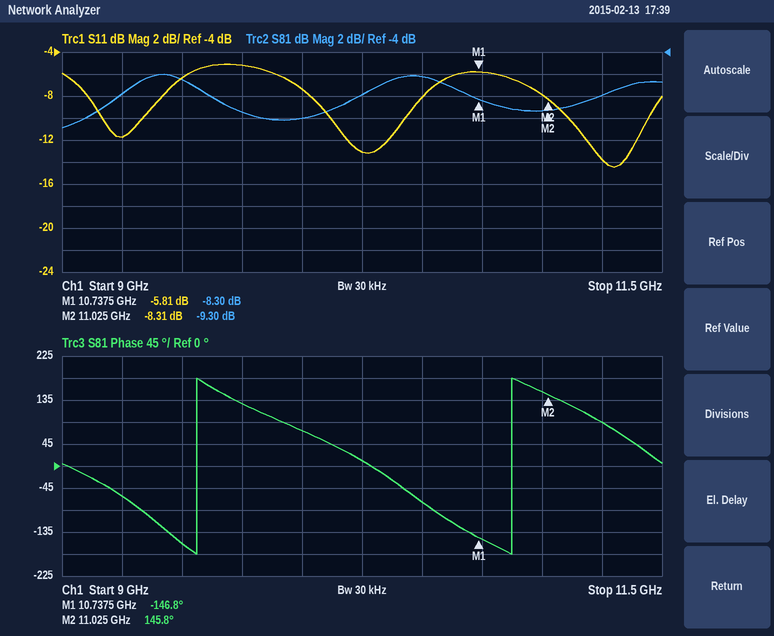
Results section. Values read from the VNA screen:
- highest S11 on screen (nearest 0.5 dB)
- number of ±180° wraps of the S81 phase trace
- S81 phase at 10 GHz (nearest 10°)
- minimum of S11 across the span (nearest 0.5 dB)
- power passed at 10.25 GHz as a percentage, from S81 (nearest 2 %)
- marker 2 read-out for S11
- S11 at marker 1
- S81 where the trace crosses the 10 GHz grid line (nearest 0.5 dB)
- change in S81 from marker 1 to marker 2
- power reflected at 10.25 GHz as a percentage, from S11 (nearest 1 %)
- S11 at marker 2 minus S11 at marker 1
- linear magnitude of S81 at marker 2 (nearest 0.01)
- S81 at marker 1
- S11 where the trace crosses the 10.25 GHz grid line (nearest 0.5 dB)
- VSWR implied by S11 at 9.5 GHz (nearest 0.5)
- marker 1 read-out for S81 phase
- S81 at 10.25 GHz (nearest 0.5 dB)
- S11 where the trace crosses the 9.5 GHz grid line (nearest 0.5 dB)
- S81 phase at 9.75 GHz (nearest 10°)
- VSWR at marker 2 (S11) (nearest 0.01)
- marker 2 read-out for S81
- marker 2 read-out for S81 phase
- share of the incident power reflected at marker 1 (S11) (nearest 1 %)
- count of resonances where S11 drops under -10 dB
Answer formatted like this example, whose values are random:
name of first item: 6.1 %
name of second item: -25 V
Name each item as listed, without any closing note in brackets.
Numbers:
highest S11 on screen: -5.0 dB
number of ±180° wraps of the S81 phase trace: 2
S81 phase at 10 GHz: 70°
minimum of S11 across the span: -14.5 dB
power passed at 10.25 GHz as a percentage, from S81: 16 %
marker 2 read-out for S11: -8.31 dB
S11 at marker 1: -5.81 dB
S81 where the trace crosses the 10 GHz grid line: -10.0 dB
change in S81 from marker 1 to marker 2: -1.00 dB
power reflected at 10.25 GHz as a percentage, from S11: 5 %
S11 at marker 2 minus S11 at marker 1: -2.50 dB
linear magnitude of S81 at marker 2: 0.34
S81 at marker 1: -8.30 dB
S11 where the trace crosses the 10.25 GHz grid line: -13.0 dB
VSWR implied by S11 at 9.5 GHz: 3.0
marker 1 read-out for S81 phase: -146.8°
S81 at 10.25 GHz: -8.0 dB
S11 where the trace crosses the 9.5 GHz grid line: -6.5 dB
S81 phase at 9.75 GHz: 130°
VSWR at marker 2 (S11): 2.25
marker 2 read-out for S81: -9.30 dB
marker 2 read-out for S81 phase: 145.8°
share of the incident power reflected at marker 1 (S11): 26 %
count of resonances where S11 drops under -10 dB: 3
